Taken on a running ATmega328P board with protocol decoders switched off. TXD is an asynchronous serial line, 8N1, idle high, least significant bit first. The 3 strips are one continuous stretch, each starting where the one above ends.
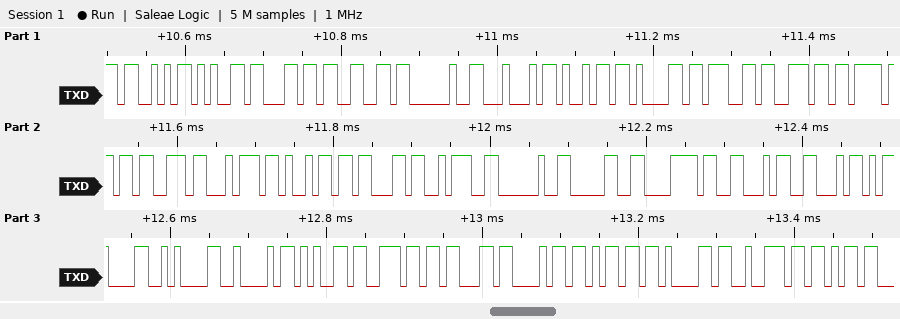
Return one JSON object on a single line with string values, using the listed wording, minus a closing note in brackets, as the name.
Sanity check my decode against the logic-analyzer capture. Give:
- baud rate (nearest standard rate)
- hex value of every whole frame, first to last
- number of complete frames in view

{"baud rate": "115200 baud", "hex value of every whole frame, first to last": "53 65 6C 66 20 44 69 61 67 6E 6F 73 74 69 63 3A 20 30 78 46 46 0D 0A 42 65 6E 63 68 6D 61 72 6B", "number of complete frames in view": "32"}
